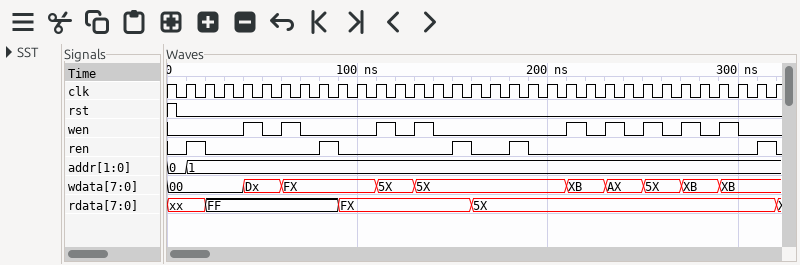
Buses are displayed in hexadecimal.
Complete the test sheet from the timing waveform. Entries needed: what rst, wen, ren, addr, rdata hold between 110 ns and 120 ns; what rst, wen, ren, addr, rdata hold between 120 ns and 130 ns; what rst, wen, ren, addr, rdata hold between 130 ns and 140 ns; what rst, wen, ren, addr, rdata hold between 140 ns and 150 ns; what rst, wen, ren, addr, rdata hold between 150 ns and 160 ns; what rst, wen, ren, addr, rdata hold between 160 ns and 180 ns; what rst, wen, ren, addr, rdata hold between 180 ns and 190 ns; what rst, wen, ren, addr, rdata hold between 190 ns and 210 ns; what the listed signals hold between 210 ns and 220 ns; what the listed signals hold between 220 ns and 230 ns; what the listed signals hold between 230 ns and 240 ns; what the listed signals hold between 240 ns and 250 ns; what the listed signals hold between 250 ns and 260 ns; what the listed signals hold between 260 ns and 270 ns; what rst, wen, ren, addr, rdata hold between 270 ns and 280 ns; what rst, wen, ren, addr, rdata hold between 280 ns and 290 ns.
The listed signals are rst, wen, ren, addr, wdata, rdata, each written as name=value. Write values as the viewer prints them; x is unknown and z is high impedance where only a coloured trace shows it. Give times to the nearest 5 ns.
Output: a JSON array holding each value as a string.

["rst=0, wen=1, ren=0, addr=1, rdata=FX", "rst=0, wen=0, ren=0, addr=1, rdata=FX", "rst=0, wen=1, ren=0, addr=1, rdata=FX", "rst=0, wen=0, ren=0, addr=1, rdata=FX", "rst=0, wen=0, ren=1, addr=1, rdata=FX", "rst=0, wen=0, ren=0, addr=1, rdata=5X", "rst=0, wen=0, ren=1, addr=1, rdata=5X", "rst=0, wen=0, ren=0, addr=1, rdata=5X", "rst=0, wen=1, ren=0, addr=1, wdata=XB, rdata=5X", "rst=0, wen=0, ren=0, addr=1, wdata=XB, rdata=5X", "rst=0, wen=1, ren=0, addr=1, wdata=AX, rdata=5X", "rst=0, wen=0, ren=0, addr=1, wdata=AX, rdata=5X", "rst=0, wen=1, ren=0, addr=1, wdata=5X, rdata=5X", "rst=0, wen=0, ren=0, addr=1, wdata=5X, rdata=5X", "rst=0, wen=1, ren=0, addr=1, rdata=5X", "rst=0, wen=0, ren=0, addr=1, rdata=5X"]
